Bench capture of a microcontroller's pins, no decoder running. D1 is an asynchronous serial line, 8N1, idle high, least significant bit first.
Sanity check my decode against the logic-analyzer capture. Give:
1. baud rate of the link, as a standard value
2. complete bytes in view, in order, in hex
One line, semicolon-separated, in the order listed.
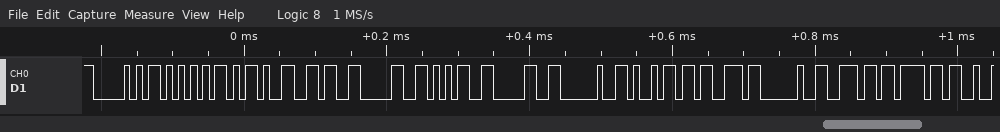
115200 baud; 0x50 0x55 0x2D 0x36 0x30 0x35 0x30 0x20 0x69 0x73 0x20 0x6E 0x6F
